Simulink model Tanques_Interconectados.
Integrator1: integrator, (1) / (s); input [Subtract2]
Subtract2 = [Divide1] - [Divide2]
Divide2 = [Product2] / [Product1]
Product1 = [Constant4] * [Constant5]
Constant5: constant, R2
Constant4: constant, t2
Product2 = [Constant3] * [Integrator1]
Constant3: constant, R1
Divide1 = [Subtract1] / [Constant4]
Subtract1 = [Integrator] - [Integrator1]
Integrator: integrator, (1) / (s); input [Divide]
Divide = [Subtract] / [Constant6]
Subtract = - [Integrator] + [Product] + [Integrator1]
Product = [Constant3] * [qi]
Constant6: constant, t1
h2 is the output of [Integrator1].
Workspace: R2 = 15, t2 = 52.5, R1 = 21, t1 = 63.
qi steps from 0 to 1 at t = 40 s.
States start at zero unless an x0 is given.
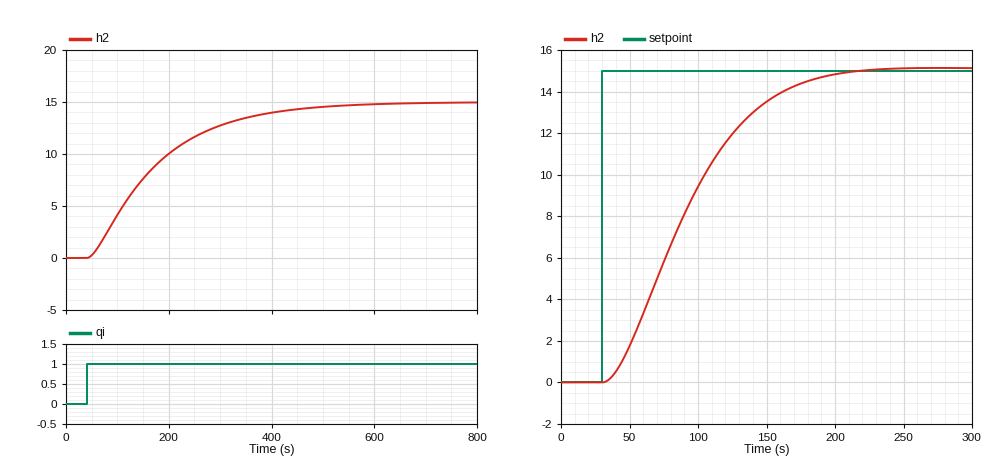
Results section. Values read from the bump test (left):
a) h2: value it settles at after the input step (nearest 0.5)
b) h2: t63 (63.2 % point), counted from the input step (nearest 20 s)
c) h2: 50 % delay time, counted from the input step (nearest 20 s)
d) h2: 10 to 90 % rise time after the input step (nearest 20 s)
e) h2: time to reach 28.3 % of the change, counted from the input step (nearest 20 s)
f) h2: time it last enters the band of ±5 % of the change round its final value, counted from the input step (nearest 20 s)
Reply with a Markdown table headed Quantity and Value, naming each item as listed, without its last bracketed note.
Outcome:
| Quantity | Value |
|---|---|
| h2: value it settles at after the input step | 15.0 |
| h2: t63 (63.2 % point), counted from the input step | 140 s |
| h2: 50 % delay time, counted from the input step | 100 s |
| h2: 10 to 90 % rise time after the input step | 280 s |
| h2: time to reach 28.3 % of the change, counted from the input step | 60 s |
| h2: time it last enters the band of ±5 % of the change round its final value, counted from the input step | 400 s |
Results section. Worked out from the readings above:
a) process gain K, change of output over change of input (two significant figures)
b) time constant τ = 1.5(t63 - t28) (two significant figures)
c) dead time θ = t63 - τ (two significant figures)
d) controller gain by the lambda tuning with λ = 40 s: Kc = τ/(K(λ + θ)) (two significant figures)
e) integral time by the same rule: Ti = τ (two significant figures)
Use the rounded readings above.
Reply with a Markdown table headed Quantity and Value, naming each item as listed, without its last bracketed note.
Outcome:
| Quantity | Value |
|---|---|
| process gain K, change of output over change of input | 15 |
| time constant τ = 1.5(t63 - t28) | 120 s |
| dead time θ = t63 - τ | 20 s |
| controller gain by the lambda tuning with λ = 40 s: Kc = τ/(K(λ + θ)) | 0.13 |
| integral time by the same rule: Ti = τ | 120 s |
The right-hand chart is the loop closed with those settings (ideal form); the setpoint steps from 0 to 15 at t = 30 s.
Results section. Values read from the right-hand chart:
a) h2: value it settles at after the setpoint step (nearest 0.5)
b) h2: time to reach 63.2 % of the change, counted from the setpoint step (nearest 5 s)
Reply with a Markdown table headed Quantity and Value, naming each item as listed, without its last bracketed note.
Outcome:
| Quantity | Value |
|---|---|
| h2: value it settles at after the setpoint step | 15.0 |
| h2: time to reach 63.2 % of the change, counted from the setpoint step | 70 s |
